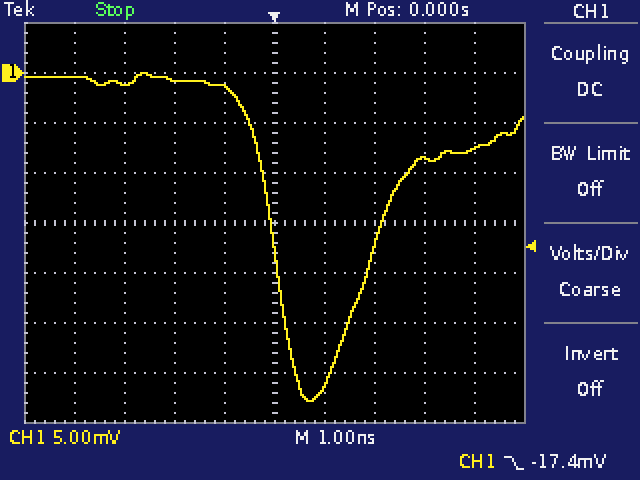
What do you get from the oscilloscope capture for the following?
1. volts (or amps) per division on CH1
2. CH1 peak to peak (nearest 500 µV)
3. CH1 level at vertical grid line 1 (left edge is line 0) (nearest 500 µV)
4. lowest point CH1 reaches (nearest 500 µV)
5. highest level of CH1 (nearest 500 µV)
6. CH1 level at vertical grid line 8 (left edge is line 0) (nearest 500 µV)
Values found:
5 mV
33.0 mV
-500 µV
-33.0 mV
0.0 mV
-8.5 mV
